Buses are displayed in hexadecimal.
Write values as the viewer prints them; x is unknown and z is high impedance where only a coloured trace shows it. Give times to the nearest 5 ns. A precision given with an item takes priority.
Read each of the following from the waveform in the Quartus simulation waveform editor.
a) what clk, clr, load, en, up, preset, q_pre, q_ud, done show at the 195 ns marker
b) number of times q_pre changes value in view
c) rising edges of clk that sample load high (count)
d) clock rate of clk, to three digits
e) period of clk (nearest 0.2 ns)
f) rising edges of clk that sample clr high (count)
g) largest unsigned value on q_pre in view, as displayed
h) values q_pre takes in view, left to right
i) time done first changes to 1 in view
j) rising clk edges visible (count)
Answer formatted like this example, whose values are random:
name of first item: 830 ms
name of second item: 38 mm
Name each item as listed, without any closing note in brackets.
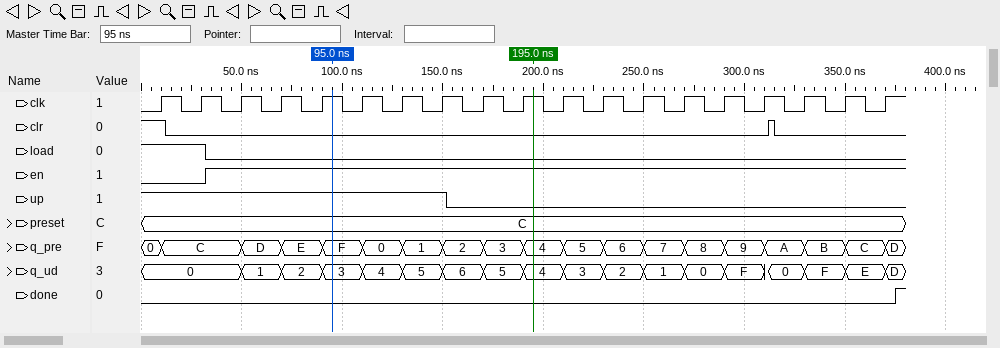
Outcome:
what clk, clr, load, en, up, preset, q_pre, q_ud, done show at the 195 ns marker: clk=1, clr=0, load=0, en=1, up=0, preset=C, q_pre=4, q_ud=4, done=0
number of times q_pre changes value in view: 18
rising edges of clk that sample load high: 2
clock rate of clk, to three digits: 50.0 MHz
period of clk: 20 ns
rising edges of clk that sample clr high: 1
largest unsigned value on q_pre in view, as displayed: F
values q_pre takes in view, left to right: 0, C, D, E, F, 0, 1, 2, 3, 4, 5, 6, 7, 8, 9, A, B, C, D
time done first changes to 1 in view: 375 ns
rising clk edges visible: 19
